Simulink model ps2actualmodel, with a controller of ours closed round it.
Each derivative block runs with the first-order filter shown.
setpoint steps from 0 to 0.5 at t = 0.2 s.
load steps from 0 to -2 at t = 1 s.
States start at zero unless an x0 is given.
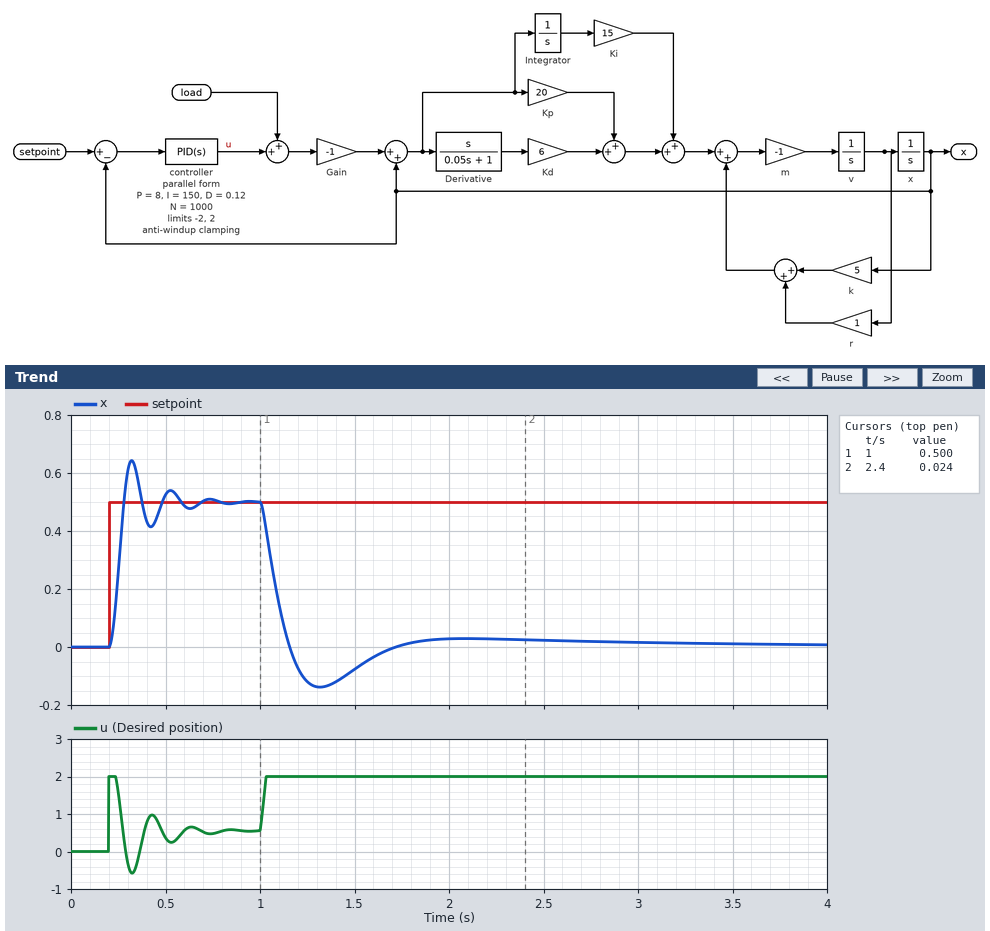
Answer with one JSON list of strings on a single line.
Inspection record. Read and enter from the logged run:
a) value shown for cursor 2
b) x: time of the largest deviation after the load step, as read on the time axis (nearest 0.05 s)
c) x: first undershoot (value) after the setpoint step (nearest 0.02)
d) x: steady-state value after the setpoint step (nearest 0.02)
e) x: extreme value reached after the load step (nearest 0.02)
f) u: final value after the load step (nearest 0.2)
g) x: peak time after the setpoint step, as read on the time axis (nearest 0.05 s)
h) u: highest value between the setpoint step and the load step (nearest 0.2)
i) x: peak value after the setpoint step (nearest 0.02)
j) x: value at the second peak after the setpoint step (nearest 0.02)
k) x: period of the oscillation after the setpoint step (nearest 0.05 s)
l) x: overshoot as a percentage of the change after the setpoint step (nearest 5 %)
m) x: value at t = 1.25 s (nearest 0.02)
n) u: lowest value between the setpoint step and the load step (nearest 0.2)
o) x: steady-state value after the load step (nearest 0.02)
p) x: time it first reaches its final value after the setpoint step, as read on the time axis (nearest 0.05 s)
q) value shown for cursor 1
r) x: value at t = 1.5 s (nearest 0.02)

["0.024", "1.30 s", "0.42", "0.50", "-0.14", "2.0", "0.30 s", "2.0", "0.64", "0.54", "0.20 s", "30 %", "-0.12", "-0.6", "0.00", "0.30 s", "0.500", "-0.08"]
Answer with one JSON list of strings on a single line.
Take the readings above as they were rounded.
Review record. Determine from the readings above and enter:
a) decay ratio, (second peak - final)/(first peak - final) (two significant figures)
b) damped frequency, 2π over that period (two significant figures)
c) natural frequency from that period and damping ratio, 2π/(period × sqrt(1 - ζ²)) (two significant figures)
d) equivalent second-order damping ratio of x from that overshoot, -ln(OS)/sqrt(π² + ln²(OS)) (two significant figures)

["0.29", "31 rad/s", "34 rad/s", "0.36"]
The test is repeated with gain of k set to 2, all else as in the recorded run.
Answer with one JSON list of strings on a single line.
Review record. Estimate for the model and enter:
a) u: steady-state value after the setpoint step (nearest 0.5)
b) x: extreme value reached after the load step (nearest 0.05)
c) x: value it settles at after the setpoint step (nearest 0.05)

["0.5", "-0.10", "0.50"]
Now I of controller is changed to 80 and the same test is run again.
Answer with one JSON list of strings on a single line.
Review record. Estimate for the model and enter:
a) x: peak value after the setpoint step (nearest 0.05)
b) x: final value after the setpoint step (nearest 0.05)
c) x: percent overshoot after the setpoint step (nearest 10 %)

["0.60", "0.50", "20 %"]
